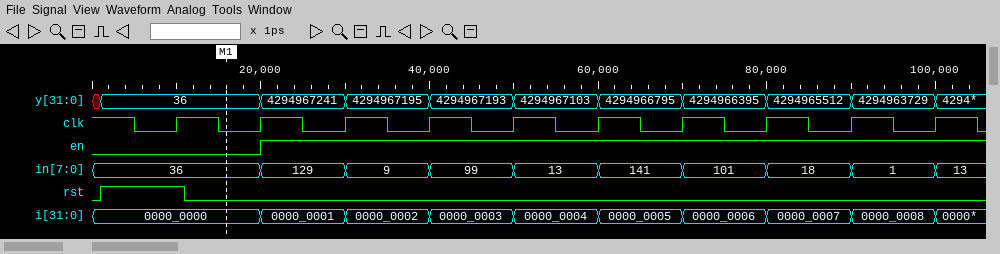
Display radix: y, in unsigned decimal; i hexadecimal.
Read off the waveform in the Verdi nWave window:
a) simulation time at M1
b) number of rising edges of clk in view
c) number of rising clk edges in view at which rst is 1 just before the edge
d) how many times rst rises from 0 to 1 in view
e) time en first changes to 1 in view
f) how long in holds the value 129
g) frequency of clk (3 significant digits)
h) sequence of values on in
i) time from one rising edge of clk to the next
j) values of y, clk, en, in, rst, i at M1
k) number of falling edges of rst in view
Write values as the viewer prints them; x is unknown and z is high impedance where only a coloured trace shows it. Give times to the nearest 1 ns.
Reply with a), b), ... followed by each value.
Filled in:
a) 16 ns
b) 10
c) 1
d) 1
e) 20 ns
f) 10 ns
g) 100 MHz
h) 36, 129, 9, 99, 13, 141, 101, 18, 1, 13
i) 10 ns
j) y=36, clk=0, en=0, in=36, rst=0, i=0000_0000
k) 1
